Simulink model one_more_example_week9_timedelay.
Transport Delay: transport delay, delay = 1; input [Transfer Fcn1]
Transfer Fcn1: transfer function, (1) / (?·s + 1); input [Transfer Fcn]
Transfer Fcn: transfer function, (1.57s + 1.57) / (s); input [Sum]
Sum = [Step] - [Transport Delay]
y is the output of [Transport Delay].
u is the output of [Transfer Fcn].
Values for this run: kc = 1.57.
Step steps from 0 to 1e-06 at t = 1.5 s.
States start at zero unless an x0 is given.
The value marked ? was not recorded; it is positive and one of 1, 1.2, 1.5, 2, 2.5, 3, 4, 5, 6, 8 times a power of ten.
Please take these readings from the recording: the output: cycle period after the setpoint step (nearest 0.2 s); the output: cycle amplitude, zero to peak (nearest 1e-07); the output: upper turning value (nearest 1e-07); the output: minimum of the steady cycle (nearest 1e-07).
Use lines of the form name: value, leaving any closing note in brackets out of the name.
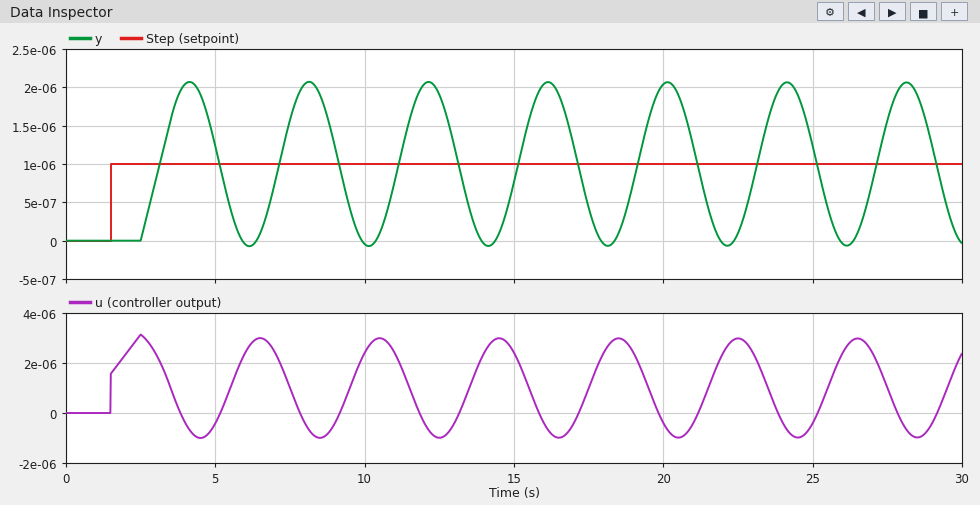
the output: cycle period after the setpoint step: 4.0 s
the output: cycle amplitude, zero to peak: 0.0000011
the output: upper turning value: 0.0000021
the output: minimum of the steady cycle: -0.0000001
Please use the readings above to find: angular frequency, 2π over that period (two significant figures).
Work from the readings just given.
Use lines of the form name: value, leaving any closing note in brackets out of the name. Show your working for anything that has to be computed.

angular frequency, 2π over that period: 2π / 4 = 1.6 rad/s
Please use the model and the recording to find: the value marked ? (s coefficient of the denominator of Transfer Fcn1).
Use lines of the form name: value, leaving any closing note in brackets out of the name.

the value marked ?: 1
